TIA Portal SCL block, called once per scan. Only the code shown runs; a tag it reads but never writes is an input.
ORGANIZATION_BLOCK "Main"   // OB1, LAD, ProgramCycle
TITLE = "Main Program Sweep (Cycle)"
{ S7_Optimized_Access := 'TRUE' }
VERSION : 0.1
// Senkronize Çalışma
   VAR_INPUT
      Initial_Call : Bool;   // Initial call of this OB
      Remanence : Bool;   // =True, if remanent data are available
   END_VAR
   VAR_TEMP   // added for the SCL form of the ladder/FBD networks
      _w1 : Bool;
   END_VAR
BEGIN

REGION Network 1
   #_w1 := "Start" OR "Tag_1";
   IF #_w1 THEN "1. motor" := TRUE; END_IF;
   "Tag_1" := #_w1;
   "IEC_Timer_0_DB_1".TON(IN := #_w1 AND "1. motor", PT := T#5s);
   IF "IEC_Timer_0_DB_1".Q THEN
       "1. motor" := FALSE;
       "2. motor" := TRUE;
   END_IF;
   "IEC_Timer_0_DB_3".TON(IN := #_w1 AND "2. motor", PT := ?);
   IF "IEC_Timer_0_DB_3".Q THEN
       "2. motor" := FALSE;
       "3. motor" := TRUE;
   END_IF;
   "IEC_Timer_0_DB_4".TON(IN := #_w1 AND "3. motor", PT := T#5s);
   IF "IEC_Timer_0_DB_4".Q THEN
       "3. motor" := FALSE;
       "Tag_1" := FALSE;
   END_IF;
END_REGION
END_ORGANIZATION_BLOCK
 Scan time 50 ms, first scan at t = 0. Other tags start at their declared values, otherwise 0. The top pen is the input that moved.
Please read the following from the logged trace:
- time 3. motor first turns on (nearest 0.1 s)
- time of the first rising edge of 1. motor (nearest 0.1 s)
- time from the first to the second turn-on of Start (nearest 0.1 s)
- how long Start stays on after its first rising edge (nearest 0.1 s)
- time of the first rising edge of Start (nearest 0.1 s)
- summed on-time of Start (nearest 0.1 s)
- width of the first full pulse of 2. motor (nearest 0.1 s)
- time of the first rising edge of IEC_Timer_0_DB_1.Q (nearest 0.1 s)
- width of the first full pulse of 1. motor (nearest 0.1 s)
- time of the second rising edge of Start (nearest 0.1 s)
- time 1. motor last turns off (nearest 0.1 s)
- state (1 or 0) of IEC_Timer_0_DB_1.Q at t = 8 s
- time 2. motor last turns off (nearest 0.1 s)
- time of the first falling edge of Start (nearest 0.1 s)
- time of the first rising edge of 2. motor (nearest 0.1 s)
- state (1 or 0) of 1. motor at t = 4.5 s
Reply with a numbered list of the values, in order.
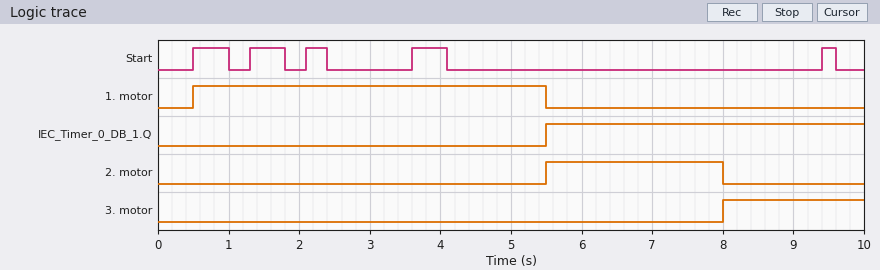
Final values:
1. 8.0 s
2. 0.5 s
3. 0.8 s
4. 0.5 s
5. 0.5 s
6. 2.0 s
7. 2.5 s
8. 5.5 s
9. 5.0 s
10. 1.3 s
11. 5.5 s
12. 1
13. 8.0 s
14. 1.0 s
15. 5.5 s
16. 1
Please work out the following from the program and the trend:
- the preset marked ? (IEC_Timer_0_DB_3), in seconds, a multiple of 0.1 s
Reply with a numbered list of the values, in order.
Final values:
1. 2.5 s
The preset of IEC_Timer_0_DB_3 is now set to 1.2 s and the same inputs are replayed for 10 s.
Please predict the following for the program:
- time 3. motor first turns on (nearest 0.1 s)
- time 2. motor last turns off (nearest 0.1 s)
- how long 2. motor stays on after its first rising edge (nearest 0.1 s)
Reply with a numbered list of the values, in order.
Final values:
1. 6.7 s
2. 6.7 s
3. 1.2 s
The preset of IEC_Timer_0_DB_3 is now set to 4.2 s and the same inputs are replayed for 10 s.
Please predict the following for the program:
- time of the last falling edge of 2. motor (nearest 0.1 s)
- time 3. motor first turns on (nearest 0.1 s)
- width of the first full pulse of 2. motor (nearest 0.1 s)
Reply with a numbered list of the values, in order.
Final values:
1. 9.7 s
2. 9.7 s
3. 4.2 s
